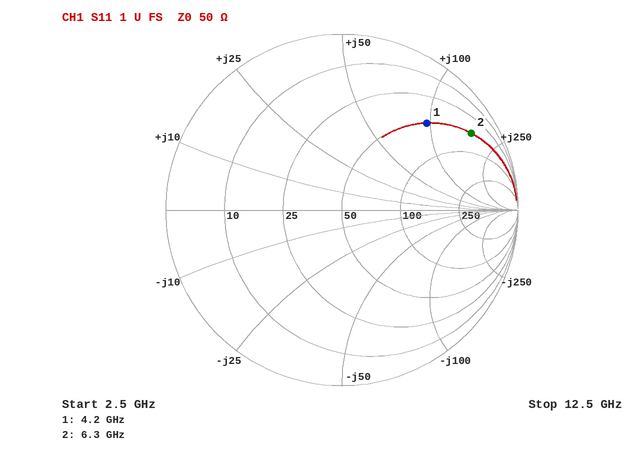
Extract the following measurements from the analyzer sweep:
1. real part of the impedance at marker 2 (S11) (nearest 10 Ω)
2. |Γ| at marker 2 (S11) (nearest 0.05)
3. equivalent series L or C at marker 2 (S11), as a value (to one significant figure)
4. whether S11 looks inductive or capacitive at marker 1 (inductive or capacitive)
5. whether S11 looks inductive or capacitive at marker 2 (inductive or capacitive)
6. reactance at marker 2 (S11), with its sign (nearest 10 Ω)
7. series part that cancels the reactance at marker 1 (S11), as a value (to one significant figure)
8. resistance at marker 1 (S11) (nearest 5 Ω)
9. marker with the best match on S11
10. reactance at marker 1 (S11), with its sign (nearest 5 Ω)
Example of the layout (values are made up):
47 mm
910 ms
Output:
50 Ω
0.85
4 nH
inductive
inductive
+170 Ω
400 fF
50 Ω
marker 1
+95 Ω
